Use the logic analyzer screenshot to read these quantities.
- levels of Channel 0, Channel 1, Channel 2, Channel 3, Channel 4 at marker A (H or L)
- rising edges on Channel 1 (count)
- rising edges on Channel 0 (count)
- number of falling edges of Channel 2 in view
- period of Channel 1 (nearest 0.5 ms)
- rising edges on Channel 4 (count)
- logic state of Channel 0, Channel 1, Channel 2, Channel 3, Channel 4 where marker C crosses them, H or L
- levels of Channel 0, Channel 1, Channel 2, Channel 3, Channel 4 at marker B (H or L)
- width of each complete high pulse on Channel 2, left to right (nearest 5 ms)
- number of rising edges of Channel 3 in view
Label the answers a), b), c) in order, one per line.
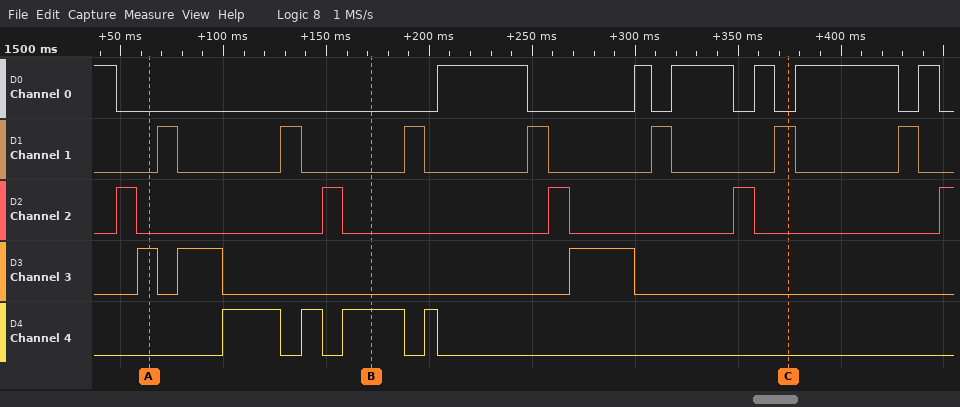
a) Channel 0=L, Channel 1=L, Channel 2=L, Channel 3=H, Channel 4=L
b) 7
c) 6
d) 4
e) 60 ms
f) 4
g) Channel 0=L, Channel 1=H, Channel 2=L, Channel 3=L, Channel 4=L
h) Channel 0=L, Channel 1=L, Channel 2=L, Channel 3=L, Channel 4=H
i) 10 ms, 10 ms, 10 ms, 10 ms
j) 3
